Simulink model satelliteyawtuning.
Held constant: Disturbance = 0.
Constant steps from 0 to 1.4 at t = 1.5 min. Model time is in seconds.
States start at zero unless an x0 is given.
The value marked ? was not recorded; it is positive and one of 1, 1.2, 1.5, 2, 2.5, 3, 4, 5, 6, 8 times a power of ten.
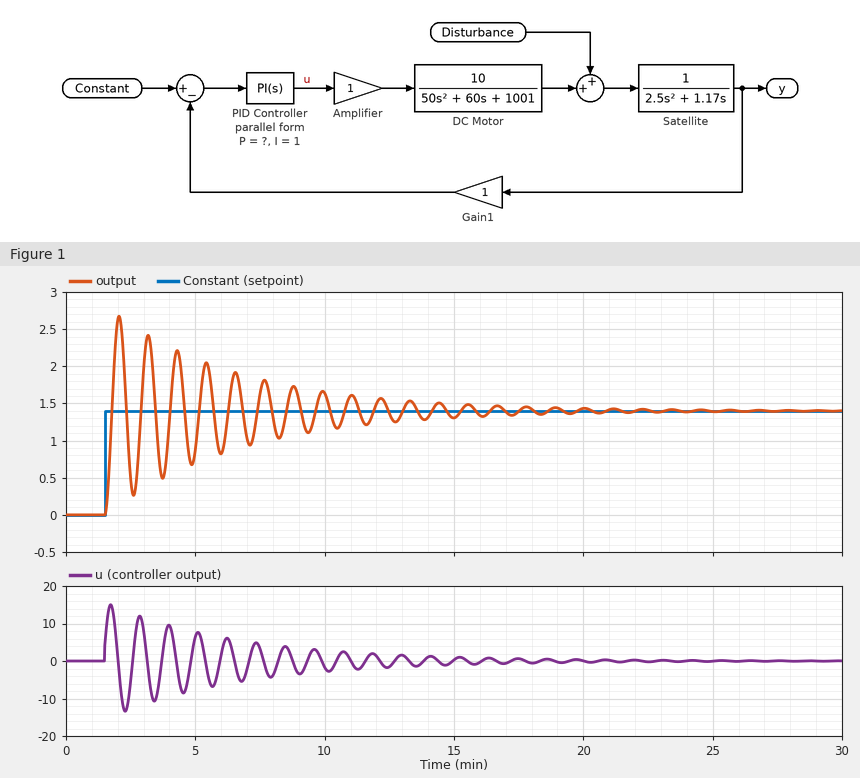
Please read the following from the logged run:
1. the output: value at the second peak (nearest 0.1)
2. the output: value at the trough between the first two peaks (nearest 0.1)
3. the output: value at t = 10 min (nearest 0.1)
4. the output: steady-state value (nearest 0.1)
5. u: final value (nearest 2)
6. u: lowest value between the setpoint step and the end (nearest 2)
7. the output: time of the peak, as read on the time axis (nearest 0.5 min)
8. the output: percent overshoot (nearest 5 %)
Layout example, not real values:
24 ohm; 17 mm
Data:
2.4; 0.3; 1.6; 1.4; 0; -14; 2.0 min; 90 %
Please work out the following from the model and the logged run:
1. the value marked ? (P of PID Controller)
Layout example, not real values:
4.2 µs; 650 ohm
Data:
3
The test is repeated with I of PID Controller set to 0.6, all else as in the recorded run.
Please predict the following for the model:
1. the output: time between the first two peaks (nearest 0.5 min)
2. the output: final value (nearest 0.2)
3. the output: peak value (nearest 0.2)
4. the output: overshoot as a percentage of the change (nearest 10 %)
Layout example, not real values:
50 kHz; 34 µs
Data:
1.5 min; 1.4; 2.4; 80 %
